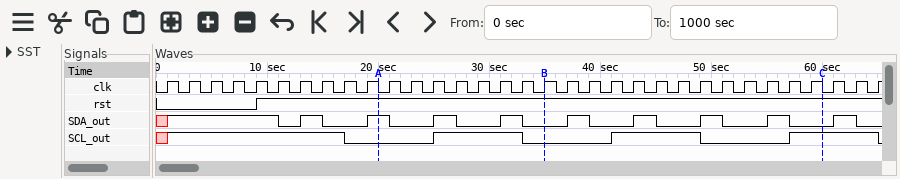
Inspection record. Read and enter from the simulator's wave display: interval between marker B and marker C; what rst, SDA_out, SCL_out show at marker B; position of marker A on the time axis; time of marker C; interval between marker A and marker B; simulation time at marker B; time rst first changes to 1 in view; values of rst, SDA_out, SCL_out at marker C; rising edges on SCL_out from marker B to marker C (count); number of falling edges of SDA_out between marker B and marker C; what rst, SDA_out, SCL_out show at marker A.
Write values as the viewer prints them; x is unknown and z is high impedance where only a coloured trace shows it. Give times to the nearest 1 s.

25 s
rst=1, SDA_out=0, SCL_out=0
20 s
60 s
15 s
35 s
9 s
rst=1, SDA_out=0, SCL_out=1
2
4
rst=1, SDA_out=1, SCL_out=0
